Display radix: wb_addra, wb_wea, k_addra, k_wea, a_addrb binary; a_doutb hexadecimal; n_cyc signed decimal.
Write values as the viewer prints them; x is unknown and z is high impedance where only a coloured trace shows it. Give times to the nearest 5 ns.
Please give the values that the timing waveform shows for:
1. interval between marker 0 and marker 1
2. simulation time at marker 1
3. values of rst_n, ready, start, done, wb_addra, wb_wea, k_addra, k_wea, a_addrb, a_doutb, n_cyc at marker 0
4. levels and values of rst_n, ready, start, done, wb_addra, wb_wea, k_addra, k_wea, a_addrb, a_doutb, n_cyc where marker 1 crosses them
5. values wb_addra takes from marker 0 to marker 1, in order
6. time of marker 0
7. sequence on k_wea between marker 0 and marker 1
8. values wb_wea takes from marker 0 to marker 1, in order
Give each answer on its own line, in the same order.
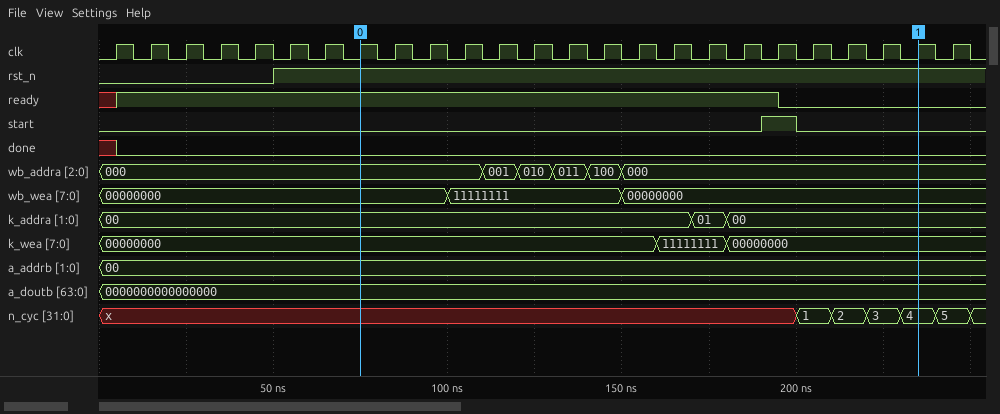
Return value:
160 ns
235 ns
rst_n=1, ready=1, start=0, done=0, wb_addra=000, wb_wea=00000000, k_addra=00, k_wea=00000000, a_addrb=00, a_doutb=0000000000000000, n_cyc=x
rst_n=1, ready=0, start=0, done=0, wb_addra=000, wb_wea=00000000, k_addra=00, k_wea=00000000, a_addrb=00, a_doutb=0000000000000000, n_cyc=4
000, 001, 010, 011, 100, 000
75 ns
00000000, 11111111, 00000000
00000000, 11111111, 00000000
